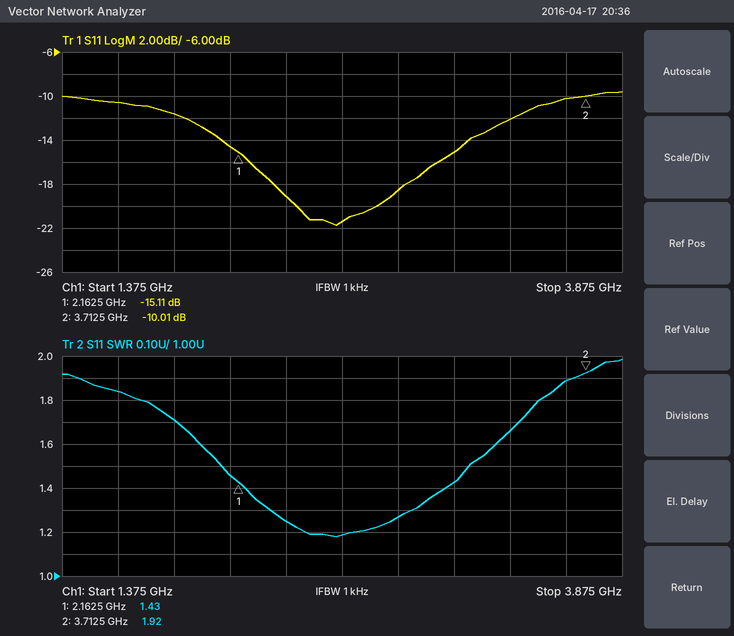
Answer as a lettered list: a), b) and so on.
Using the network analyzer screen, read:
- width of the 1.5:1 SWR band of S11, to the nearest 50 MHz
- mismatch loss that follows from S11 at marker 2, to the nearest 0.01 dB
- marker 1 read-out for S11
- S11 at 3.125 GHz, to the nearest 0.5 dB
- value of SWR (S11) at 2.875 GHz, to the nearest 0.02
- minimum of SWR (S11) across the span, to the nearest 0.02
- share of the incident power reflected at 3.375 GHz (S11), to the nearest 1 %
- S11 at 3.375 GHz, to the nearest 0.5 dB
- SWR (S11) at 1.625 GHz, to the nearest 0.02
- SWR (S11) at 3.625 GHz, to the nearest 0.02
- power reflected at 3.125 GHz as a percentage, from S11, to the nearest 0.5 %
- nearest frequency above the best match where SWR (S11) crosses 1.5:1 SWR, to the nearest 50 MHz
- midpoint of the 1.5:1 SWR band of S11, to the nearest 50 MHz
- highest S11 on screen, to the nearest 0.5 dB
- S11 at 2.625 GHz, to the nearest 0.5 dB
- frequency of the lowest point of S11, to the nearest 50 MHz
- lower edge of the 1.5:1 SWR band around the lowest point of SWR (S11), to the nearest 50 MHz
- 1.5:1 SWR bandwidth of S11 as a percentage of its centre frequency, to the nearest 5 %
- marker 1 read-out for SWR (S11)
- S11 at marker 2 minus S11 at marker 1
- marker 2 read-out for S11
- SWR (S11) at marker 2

a) 1.10 GHz
b) 0.46 dB
c) -15.11 dB
d) -15.0 dB
e) 1.26
f) 1.18
g) 6 %
h) -12.0 dB
i) 1.84
j) 1.88
k) 3.0 %
l) 3.20 GHz
m) 2.65 GHz
n) -9.5 dB
o) -21.5 dB
p) 2.60 GHz
q) 2.10 GHz
r) 40 %
s) 1.43
t) 5.10 dB
u) -10.01 dB
v) 1.92
